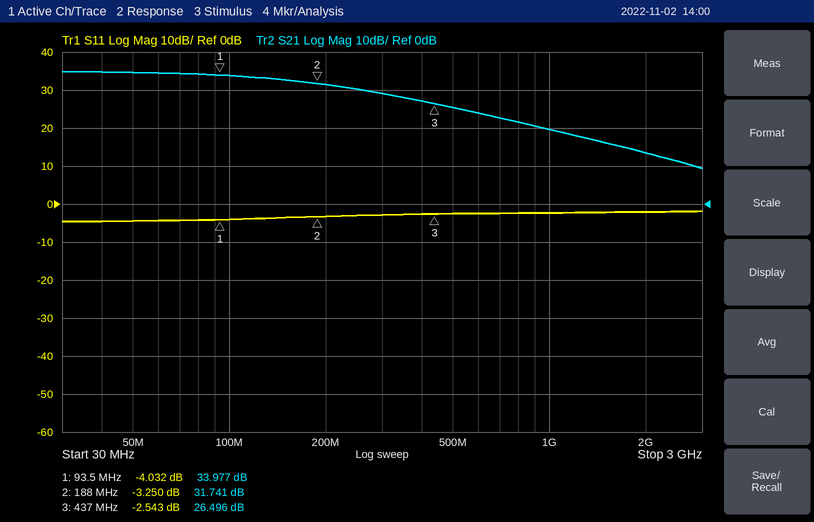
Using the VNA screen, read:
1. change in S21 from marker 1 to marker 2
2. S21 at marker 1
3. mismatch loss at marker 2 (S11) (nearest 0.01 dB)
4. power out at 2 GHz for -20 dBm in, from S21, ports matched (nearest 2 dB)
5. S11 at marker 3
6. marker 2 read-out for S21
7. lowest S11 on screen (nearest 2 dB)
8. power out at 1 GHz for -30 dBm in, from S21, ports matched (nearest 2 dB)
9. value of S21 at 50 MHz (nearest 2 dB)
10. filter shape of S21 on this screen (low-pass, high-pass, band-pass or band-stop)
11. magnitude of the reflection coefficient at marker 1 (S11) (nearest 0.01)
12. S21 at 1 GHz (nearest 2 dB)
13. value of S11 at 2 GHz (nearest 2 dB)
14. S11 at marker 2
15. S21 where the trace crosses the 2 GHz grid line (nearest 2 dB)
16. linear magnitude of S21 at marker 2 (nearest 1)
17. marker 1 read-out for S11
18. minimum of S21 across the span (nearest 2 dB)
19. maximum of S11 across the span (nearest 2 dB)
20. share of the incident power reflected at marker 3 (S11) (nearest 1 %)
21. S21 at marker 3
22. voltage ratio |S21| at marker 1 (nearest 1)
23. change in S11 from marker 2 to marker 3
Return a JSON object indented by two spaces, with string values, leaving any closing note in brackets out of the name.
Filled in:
{
  "change in S21 from marker 1 to marker 2": "-2.236 dB",
  "S21 at marker 1": "33.977 dB",
  "mismatch loss at marker 2 (S11)": "2.78 dB",
  "power out at 2 GHz for -20 dBm in, from S21, ports matched": "-6 dBm",
  "S11 at marker 3": "-2.543 dB",
  "marker 2 read-out for S21": "31.741 dB",
  "lowest S11 on screen": "-4 dB",
  "power out at 1 GHz for -30 dBm in, from S21, ports matched": "-10 dBm",
  "value of S21 at 50 MHz": "34 dB",
  "filter shape of S21 on this screen": "low-pass",
  "magnitude of the reflection coefficient at marker 1 (S11)": "0.63",
  "S21 at 1 GHz": "20 dB",
  "value of S11 at 2 GHz": "-2 dB",
  "S11 at marker 2": "-3.250 dB",
  "S21 where the trace crosses the 2 GHz grid line": "14 dB",
  "linear magnitude of S21 at marker 2": "39",
  "marker 1 read-out for S11": "-4.032 dB",
  "minimum of S21 across the span": "10 dB",
  "maximum of S11 across the span": "-2 dB",
  "share of the incident power reflected at marker 3 (S11)": "56 %",
  "S21 at marker 3": "26.496 dB",
  "voltage ratio |S21| at marker 1": "50",
  "change in S11 from marker 2 to marker 3": "0.707 dB"
}
